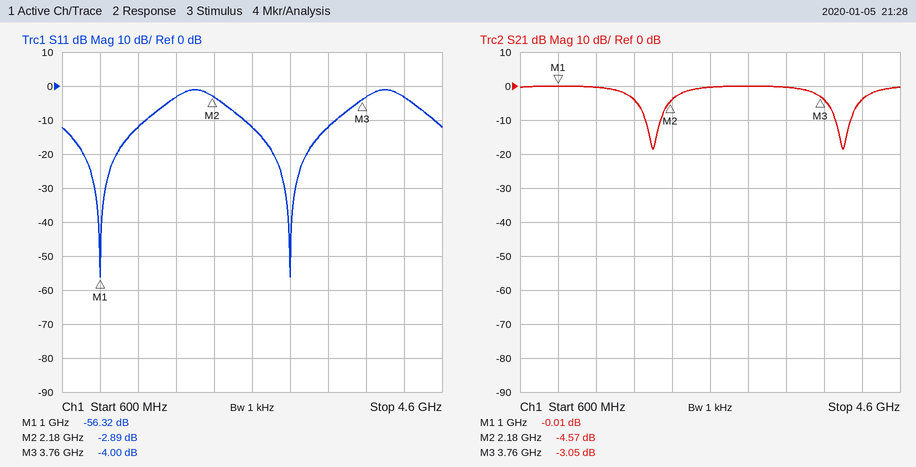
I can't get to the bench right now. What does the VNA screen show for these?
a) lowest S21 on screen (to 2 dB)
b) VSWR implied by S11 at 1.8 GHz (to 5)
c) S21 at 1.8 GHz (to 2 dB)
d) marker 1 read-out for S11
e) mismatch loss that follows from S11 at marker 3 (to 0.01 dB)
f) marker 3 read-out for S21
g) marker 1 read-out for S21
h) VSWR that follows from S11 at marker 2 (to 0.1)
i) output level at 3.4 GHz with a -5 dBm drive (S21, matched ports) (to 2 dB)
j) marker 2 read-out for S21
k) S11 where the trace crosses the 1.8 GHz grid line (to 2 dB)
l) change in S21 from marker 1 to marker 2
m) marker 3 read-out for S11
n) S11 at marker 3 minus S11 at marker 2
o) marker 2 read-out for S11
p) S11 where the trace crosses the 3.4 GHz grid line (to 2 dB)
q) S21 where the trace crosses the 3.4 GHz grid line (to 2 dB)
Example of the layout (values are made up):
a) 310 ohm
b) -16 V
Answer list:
a) -18 dB
b) 5
c) -4 dB
d) -56.32 dB
e) 2.20 dB
f) -3.05 dB
g) -0.01 dB
h) 6.1
i) -6 dBm
j) -4.57 dB
k) -4 dB
l) -4.56 dB
m) -4.00 dB
n) -1.11 dB
o) -2.89 dB
p) -12 dB
q) 0 dB
